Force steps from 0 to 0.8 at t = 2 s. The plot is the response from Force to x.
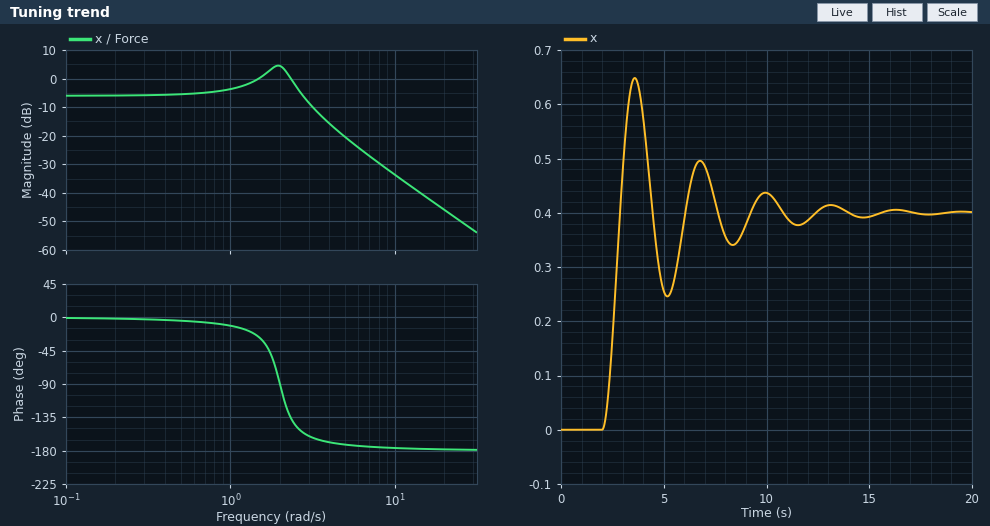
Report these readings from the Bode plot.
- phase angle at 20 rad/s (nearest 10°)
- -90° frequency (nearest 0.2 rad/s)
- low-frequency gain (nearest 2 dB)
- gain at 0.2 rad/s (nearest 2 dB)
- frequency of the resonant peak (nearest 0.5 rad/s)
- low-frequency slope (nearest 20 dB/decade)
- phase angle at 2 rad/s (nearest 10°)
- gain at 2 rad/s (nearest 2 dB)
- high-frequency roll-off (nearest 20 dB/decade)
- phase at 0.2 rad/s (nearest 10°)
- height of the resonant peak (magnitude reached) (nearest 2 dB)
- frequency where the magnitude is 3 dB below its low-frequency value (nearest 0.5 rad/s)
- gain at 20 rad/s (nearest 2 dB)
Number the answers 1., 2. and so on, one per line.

1. -180°
2. 2.0 rad/s
3. -6 dB
4. -6 dB
5. 2.0 rad/s
6. 0 dB/decade
7. -90°
8. 4 dB
9. -40 dB/decade
10. 0°
11. 4 dB
12. 3.0 rad/s
13. -46 dB
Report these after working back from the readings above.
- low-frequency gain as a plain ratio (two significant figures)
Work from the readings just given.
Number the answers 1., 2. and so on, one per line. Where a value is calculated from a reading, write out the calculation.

1. 10^(-6 / 20) = 0.50
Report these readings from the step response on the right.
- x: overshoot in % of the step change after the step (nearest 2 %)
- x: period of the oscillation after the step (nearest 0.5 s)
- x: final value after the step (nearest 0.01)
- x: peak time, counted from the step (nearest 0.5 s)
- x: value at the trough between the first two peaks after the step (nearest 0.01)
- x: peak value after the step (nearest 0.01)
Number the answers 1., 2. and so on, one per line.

1. 62 %
2. 3.0 s
3. 0.40
4. 1.5 s
5. 0.25
6. 0.65
